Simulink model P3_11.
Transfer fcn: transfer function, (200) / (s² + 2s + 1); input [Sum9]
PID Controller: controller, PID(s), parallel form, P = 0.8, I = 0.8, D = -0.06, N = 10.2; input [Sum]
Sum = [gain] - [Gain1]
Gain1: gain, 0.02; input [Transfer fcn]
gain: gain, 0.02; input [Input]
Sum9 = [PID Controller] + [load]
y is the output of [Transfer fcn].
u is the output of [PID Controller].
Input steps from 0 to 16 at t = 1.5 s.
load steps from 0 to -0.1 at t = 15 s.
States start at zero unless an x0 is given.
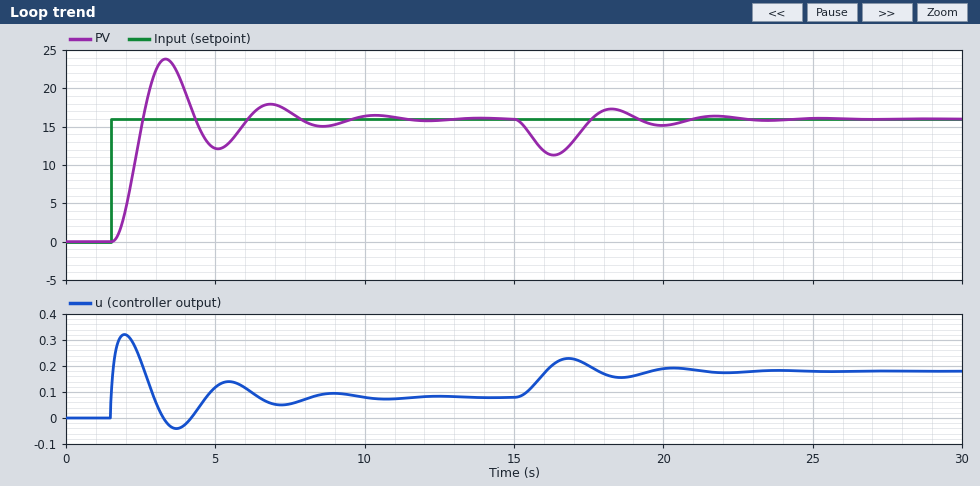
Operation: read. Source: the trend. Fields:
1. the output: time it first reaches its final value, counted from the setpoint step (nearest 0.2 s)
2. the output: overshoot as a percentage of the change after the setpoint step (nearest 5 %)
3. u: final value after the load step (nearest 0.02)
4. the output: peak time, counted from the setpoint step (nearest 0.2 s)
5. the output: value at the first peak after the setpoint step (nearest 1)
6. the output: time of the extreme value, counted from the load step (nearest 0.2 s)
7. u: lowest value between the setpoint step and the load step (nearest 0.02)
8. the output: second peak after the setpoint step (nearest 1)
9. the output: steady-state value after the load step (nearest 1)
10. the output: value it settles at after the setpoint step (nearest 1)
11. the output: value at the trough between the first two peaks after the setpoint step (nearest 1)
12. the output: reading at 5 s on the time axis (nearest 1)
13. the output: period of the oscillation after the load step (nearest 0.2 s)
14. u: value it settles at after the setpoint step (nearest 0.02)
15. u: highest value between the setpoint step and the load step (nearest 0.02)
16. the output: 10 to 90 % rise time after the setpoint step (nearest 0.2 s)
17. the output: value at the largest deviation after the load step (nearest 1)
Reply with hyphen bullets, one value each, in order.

- 1.0 s
- 50 %
- 0.18
- 1.8 s
- 24
- 1.4 s
- -0.04
- 18
- 16
- 16
- 12
- 12
- 3.6 s
- 0.08
- 0.32
- 0.6 s
- 11
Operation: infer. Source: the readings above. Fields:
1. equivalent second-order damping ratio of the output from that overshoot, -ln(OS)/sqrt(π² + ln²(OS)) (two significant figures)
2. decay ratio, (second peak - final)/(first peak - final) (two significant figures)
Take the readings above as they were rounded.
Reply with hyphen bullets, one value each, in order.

- 0.22
- 0.25
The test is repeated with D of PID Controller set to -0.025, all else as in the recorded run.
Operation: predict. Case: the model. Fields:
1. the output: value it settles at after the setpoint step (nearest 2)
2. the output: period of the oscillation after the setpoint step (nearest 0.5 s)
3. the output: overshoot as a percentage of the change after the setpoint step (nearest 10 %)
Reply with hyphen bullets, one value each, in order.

- 16
- 3.5 s
- 40 %
